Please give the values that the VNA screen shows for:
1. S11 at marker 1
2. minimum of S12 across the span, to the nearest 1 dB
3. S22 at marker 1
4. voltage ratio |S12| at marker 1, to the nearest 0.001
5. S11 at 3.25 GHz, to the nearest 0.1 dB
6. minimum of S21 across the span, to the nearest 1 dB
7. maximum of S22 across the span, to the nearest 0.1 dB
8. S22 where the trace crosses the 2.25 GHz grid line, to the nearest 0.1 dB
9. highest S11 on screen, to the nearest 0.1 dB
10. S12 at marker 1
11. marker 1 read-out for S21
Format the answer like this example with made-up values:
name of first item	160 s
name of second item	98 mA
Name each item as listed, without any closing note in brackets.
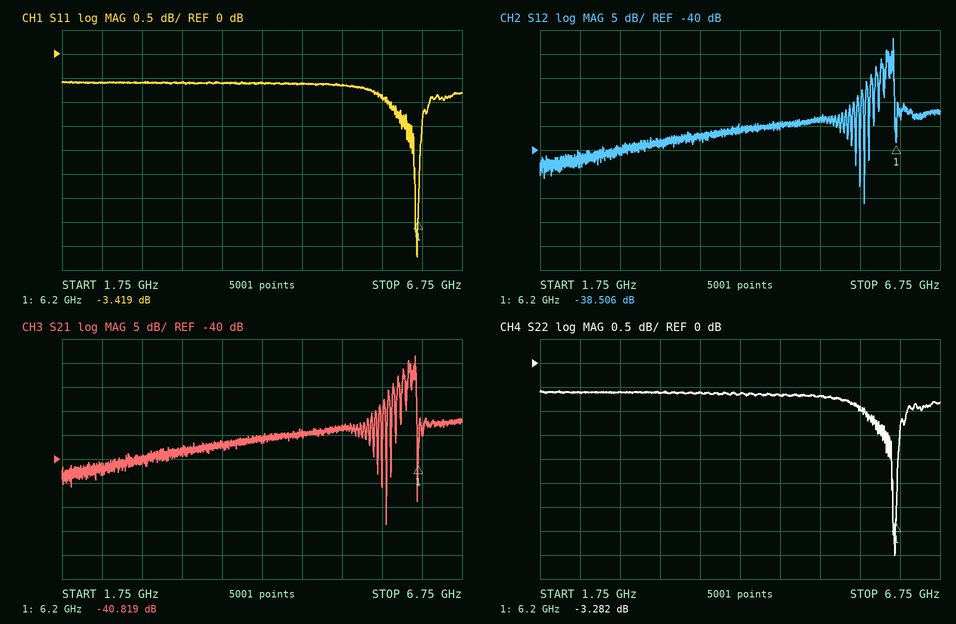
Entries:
S11 at marker 1	-3.419 dB
minimum of S12 across the span, to the nearest 1 dB	-51 dB
S22 at marker 1	-3.282 dB
voltage ratio |S12| at marker 1, to the nearest 0.001	0.012
S11 at 3.25 GHz, to the nearest 0.1 dB	-0.6 dB
minimum of S21 across the span, to the nearest 1 dB	-54 dB
maximum of S22 across the span, to the nearest 0.1 dB	-0.6 dB
S22 where the trace crosses the 2.25 GHz grid line, to the nearest 0.1 dB	-0.6 dB
highest S11 on screen, to the nearest 0.1 dB	-0.6 dB
S12 at marker 1	-38.506 dB
marker 1 read-out for S21	-40.819 dB
